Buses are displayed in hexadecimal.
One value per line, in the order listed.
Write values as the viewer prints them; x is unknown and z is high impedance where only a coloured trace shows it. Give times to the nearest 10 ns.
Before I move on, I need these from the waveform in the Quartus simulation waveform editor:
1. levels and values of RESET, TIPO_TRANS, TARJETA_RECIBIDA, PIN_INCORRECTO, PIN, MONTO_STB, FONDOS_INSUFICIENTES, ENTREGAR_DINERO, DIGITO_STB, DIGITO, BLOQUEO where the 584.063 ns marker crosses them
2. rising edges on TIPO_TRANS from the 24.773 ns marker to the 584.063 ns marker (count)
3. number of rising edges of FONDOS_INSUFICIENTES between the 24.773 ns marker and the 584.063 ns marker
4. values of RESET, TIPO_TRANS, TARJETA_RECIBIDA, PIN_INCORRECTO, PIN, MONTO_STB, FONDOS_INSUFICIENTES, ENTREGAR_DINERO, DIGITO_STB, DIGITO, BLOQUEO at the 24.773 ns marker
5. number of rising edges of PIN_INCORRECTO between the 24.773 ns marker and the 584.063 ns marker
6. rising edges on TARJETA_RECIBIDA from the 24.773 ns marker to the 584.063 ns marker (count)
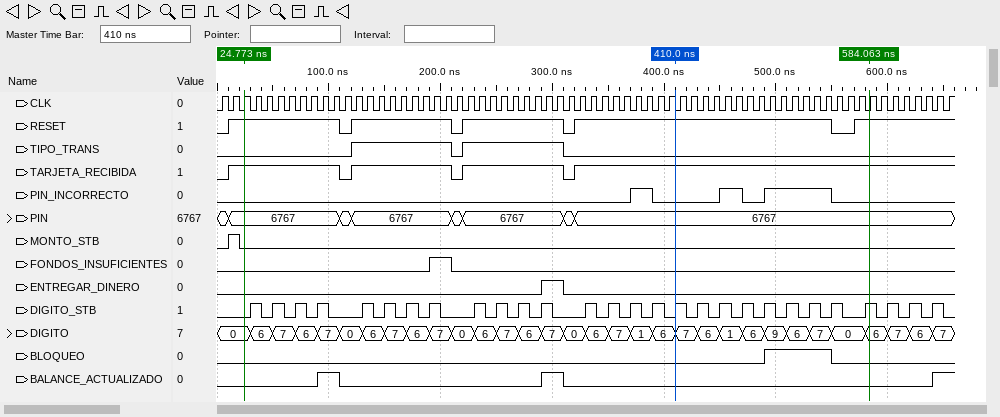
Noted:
RESET=1, TIPO_TRANS=0, TARJETA_RECIBIDA=1, PIN_INCORRECTO=0, PIN=6767, MONTO_STB=0, FONDOS_INSUFICIENTES=0, ENTREGAR_DINERO=0, DIGITO_STB=1, DIGITO=6, BLOQUEO=0
2
1
RESET=1, TIPO_TRANS=0, TARJETA_RECIBIDA=1, PIN_INCORRECTO=0, PIN=6767, MONTO_STB=0, FONDOS_INSUFICIENTES=0, ENTREGAR_DINERO=0, DIGITO_STB=0, DIGITO=0, BLOQUEO=0
3
3
